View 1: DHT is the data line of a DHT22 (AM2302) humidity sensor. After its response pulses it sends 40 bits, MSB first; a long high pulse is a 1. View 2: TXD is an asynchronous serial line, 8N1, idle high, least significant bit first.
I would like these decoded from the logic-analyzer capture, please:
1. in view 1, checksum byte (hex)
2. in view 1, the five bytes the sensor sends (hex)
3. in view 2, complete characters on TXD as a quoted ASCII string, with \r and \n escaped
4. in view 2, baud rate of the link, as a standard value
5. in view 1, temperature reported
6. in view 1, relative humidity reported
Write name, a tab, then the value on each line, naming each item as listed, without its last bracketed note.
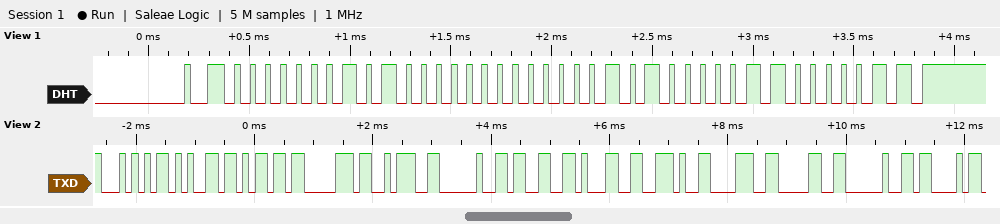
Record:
in view 1, checksum byte	0x83
in view 1, the five bytes the sensor sends	01 40 01 41 83
in view 2, complete characters on TXD as a quoted ASCII string, with \r and \n escaped	"Temp: 31.80 C"
in view 2, baud rate of the link, as a standard value	9600 baud
in view 1, temperature reported	32.1 °C
in view 1, relative humidity reported	32.0 %
